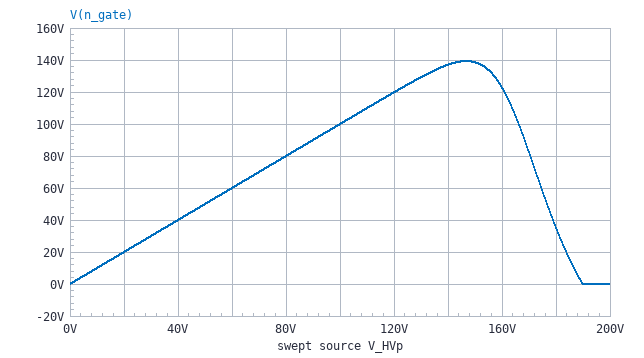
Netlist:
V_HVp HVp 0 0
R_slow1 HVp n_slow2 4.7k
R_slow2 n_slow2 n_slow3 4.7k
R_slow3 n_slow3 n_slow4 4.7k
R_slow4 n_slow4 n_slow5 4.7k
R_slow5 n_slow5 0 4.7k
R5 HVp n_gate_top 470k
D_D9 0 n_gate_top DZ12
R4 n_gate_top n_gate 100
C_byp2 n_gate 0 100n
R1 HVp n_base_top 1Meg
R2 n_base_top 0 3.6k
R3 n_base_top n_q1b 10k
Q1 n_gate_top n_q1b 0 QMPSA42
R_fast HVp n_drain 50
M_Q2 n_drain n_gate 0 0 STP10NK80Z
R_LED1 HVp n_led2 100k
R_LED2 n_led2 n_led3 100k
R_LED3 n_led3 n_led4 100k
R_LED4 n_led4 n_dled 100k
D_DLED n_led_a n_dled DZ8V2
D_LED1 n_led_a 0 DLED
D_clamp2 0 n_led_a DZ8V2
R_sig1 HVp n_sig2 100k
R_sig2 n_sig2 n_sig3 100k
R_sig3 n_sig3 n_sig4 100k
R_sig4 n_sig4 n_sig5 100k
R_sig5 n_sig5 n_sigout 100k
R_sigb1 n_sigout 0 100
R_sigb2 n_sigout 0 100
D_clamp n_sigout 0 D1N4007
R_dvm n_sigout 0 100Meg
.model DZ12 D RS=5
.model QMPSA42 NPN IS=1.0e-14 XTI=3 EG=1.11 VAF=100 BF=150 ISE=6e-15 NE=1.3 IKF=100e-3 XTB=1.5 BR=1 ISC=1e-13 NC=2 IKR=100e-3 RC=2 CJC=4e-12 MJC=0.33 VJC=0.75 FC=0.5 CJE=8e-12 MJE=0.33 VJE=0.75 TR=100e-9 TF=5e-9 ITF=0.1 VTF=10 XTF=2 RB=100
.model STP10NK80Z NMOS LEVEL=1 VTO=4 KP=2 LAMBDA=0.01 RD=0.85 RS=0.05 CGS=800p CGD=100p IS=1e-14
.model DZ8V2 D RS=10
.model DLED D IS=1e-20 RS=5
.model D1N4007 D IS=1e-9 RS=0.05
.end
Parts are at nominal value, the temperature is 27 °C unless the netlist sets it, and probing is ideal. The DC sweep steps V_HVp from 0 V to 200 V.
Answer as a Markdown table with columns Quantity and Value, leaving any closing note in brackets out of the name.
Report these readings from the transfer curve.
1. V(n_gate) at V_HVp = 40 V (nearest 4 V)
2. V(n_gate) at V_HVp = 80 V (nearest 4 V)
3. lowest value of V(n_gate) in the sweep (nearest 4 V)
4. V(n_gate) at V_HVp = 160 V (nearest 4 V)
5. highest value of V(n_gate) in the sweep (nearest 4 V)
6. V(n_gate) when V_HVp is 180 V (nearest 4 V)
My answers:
| Quantity | Value |
|---|---|
| V(n_gate) at V_HVp = 40 V | 40 V |
| V(n_gate) at V_HVp = 80 V | 80 V |
| lowest value of V(n_gate) in the sweep | 0 V |
| V(n_gate) at V_HVp = 160 V | 124 V |
| highest value of V(n_gate) in the sweep | 140 V |
| V(n_gate) when V_HVp is 180 V | 36 V |
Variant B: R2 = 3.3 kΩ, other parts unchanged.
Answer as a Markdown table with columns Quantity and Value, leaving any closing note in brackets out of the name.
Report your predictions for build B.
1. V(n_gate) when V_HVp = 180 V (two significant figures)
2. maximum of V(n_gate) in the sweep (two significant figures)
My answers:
| Quantity | Value |
|---|---|
| V(n_gate) when V_HVp = 180 V | 120 V |
| maximum of V(n_gate) in the sweep | 150 V |
